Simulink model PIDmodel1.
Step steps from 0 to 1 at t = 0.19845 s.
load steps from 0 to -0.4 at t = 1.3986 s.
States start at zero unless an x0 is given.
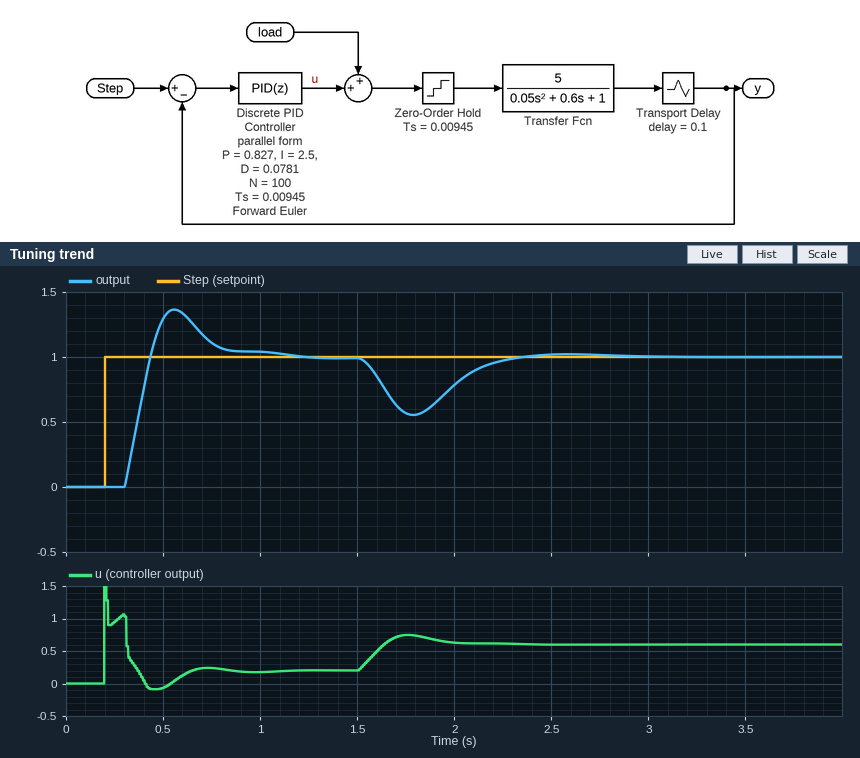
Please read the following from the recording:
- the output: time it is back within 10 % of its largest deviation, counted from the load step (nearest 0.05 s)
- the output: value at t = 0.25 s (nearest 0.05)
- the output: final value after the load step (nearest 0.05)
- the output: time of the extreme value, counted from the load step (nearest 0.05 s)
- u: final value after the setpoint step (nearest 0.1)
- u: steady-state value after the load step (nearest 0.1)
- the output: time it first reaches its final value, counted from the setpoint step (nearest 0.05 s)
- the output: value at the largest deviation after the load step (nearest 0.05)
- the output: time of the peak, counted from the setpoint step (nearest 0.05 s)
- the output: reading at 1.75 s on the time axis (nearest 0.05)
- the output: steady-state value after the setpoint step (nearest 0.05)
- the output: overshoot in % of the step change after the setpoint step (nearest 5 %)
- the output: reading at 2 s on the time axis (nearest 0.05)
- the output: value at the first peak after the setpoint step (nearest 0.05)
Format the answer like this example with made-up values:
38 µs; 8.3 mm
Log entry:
0.80 s; 0.00; 1.00; 0.40 s; 0.2; 0.6; 0.25 s; 0.55; 0.35 s; 0.55; 1.00; 35 %; 0.80; 1.35
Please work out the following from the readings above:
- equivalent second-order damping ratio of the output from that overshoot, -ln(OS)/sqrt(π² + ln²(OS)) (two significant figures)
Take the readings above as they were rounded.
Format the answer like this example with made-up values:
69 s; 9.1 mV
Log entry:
0.32
